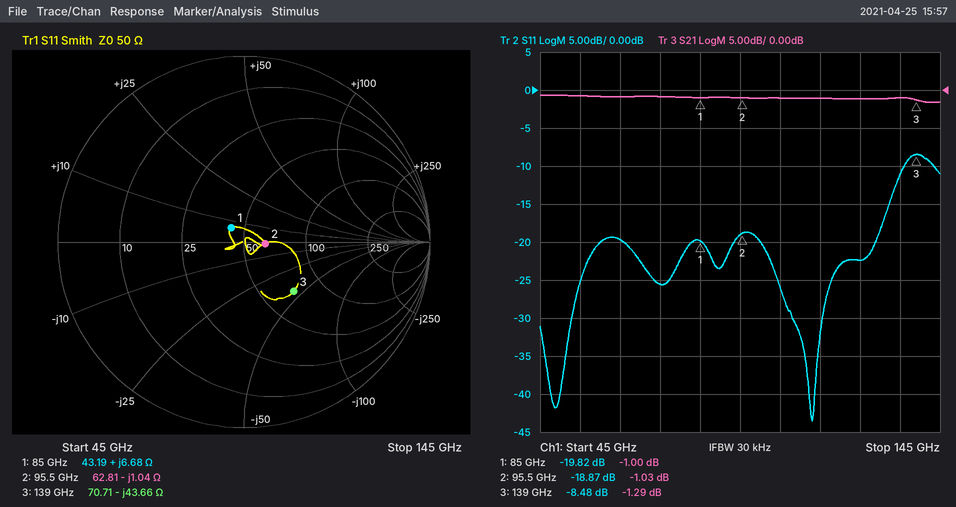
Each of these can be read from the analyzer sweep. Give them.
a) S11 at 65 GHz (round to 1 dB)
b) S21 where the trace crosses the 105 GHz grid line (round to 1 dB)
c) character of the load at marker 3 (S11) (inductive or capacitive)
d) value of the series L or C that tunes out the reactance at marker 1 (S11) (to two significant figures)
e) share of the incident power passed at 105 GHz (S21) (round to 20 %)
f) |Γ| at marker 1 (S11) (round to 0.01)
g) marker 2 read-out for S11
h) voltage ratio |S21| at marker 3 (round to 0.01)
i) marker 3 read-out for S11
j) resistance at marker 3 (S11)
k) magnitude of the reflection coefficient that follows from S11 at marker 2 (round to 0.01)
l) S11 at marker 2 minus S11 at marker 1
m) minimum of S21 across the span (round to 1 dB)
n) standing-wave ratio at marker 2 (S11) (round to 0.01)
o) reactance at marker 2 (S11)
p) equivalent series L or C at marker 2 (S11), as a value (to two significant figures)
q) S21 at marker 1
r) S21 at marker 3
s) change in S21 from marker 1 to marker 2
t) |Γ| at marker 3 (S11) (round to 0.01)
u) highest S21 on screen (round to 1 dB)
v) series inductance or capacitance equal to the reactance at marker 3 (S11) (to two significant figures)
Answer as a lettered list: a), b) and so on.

a) -20 dB
b) -1 dB
c) capacitive
d) 280 fF
e) 80 %
f) 0.10
g) -18.87 dB
h) 0.86
i) -8.48 dB
j) 70.71 Ω
k) 0.11
l) 0.95 dB
m) -2 dB
n) 1.26
o) -1.04 Ω
p) 1.6 pF
q) -1.00 dB
r) -1.29 dB
s) -0.03 dB
t) 0.38
u) -1 dB
v) 26 fF
